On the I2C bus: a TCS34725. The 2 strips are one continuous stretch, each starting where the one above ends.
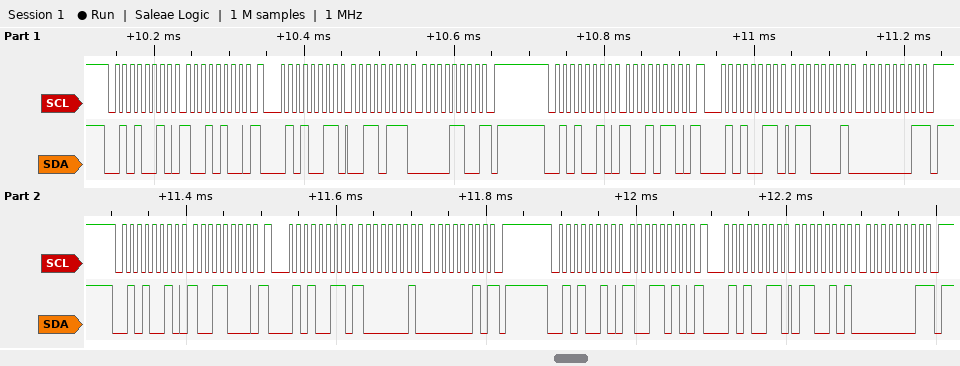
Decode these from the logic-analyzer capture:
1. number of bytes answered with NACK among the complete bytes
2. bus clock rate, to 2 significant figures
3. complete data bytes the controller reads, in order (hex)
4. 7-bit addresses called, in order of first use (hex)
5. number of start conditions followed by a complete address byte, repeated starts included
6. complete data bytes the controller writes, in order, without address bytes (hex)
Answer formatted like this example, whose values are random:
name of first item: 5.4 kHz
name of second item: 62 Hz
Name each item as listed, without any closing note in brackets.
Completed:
number of bytes answered with NACK among the complete bytes: 4
bus clock rate, to 2 significant figures: 100 kHz
complete data bytes the controller reads, in order: 37 0C 61 01 81 02 65 01
7-bit addresses called, in order of first use: 0x29
number of start conditions followed by a complete address byte, repeated starts included: 8
complete data bytes the controller writes, in order, without address bytes: 94 96 98 9A
